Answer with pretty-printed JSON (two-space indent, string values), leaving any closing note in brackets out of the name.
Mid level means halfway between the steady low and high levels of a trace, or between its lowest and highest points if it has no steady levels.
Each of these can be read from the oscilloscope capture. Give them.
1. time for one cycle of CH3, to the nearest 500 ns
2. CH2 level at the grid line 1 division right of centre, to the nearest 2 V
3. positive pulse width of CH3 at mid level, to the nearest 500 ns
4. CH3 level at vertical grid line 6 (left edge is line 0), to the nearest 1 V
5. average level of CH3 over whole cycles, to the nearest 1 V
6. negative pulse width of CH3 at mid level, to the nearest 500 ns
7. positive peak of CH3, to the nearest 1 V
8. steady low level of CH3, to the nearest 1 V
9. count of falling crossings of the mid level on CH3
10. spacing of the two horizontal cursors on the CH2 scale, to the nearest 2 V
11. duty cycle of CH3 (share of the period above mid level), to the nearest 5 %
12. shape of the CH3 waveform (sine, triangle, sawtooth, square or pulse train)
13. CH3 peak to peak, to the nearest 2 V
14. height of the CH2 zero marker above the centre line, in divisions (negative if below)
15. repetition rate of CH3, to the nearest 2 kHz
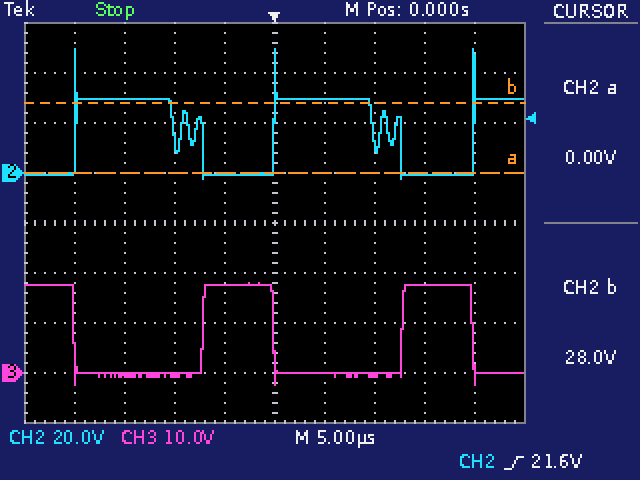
{
  "time for one cycle of CH3, to the nearest 500 ns": "20.0 µs",
  "CH2 level at the grid line 1 division right of centre, to the nearest 2 V": "30 V",
  "positive pulse width of CH3 at mid level, to the nearest 500 ns": "7.0 µs",
  "CH3 level at vertical grid line 6 (left edge is line 0), to the nearest 1 V": "0 V",
  "average level of CH3 over whole cycles, to the nearest 1 V": "6 V",
  "negative pulse width of CH3 at mid level, to the nearest 500 ns": "13.0 µs",
  "positive peak of CH3, to the nearest 1 V": "18 V",
  "steady low level of CH3, to the nearest 1 V": "0 V",
  "count of falling crossings of the mid level on CH3": "3",
  "spacing of the two horizontal cursors on the CH2 scale, to the nearest 2 V": "28 V",
  "duty cycle of CH3 (share of the period above mid level), to the nearest 5 %": "35 %",
  "shape of the CH3 waveform": "pulse train",
  "CH3 peak to peak, to the nearest 2 V": "20 V",
  "height of the CH2 zero marker above the centre line, in divisions": "+1.0 div",
  "repetition rate of CH3, to the nearest 2 kHz": "50 kHz"
}
